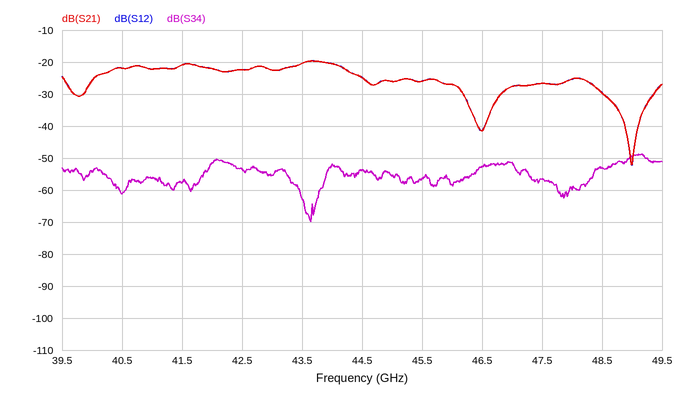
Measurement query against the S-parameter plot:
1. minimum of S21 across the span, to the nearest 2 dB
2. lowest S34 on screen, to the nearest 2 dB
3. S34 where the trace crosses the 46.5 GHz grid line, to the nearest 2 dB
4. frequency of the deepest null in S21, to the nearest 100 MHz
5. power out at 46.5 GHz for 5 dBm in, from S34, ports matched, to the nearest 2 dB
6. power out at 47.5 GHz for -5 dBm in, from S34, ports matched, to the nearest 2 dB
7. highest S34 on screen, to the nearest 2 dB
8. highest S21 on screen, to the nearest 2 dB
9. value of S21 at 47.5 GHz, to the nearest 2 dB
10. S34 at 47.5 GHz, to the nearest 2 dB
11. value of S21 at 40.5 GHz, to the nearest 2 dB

-52 dB
-70 dB
-52 dB
49.0 GHz
-48 dBm
-62 dBm
-48 dB
-20 dB
-26 dB
-56 dB
-22 dB
